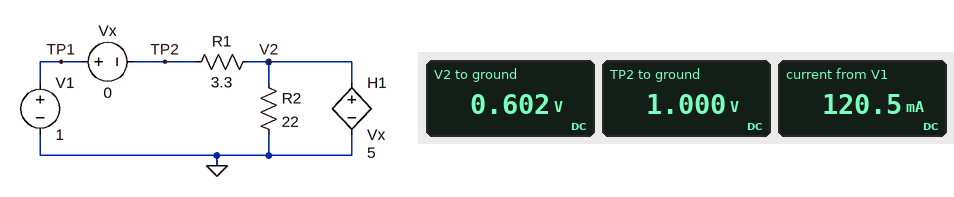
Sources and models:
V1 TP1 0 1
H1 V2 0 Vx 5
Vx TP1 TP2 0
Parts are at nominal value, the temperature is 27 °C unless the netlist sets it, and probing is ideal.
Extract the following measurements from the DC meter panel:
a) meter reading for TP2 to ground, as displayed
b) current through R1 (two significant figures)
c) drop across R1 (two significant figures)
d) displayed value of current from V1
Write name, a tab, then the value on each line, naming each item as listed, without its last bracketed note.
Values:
meter reading for TP2 to ground, as displayed	1.000 V
current through R1	120 mA
drop across R1	400 mV
displayed value of current from V1	120.5 mA
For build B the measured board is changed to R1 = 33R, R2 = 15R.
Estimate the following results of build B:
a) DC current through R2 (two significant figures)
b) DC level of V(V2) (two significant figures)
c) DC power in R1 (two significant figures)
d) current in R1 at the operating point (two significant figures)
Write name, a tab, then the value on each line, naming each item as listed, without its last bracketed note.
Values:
DC current through R2	8.8 mA
DC level of V(V2)	130 mV
DC power in R1	23 mW
current in R1 at the operating point	26 mA
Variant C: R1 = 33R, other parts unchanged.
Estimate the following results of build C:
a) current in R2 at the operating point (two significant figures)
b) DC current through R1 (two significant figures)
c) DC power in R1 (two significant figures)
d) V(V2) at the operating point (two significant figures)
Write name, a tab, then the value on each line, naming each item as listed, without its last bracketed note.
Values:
current in R2 at the operating point	6.0 mA
DC current through R1	26 mA
DC power in R1	23 mW
V(V2) at the operating point	130 mV
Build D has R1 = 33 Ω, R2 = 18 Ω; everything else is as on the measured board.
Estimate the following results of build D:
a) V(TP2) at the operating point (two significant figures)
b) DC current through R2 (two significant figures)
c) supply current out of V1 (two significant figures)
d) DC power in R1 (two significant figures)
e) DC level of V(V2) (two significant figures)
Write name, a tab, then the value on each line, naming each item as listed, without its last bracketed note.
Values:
V(TP2) at the operating point	1.0 V
DC current through R2	7.3 mA
supply current out of V1	26 mA
DC power in R1	23 mW
DC level of V(V2)	130 mV
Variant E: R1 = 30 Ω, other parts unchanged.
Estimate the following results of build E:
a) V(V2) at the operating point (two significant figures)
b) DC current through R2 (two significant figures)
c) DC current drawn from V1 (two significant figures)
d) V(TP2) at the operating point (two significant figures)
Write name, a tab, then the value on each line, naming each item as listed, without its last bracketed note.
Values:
V(V2) at the operating point	140 mV
DC current through R2	6.5 mA
DC current drawn from V1	29 mA
V(TP2) at the operating point	1.0 V
